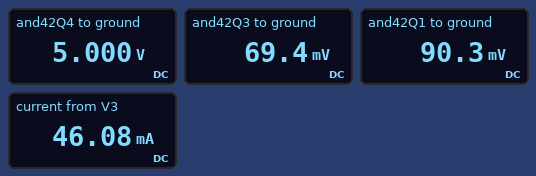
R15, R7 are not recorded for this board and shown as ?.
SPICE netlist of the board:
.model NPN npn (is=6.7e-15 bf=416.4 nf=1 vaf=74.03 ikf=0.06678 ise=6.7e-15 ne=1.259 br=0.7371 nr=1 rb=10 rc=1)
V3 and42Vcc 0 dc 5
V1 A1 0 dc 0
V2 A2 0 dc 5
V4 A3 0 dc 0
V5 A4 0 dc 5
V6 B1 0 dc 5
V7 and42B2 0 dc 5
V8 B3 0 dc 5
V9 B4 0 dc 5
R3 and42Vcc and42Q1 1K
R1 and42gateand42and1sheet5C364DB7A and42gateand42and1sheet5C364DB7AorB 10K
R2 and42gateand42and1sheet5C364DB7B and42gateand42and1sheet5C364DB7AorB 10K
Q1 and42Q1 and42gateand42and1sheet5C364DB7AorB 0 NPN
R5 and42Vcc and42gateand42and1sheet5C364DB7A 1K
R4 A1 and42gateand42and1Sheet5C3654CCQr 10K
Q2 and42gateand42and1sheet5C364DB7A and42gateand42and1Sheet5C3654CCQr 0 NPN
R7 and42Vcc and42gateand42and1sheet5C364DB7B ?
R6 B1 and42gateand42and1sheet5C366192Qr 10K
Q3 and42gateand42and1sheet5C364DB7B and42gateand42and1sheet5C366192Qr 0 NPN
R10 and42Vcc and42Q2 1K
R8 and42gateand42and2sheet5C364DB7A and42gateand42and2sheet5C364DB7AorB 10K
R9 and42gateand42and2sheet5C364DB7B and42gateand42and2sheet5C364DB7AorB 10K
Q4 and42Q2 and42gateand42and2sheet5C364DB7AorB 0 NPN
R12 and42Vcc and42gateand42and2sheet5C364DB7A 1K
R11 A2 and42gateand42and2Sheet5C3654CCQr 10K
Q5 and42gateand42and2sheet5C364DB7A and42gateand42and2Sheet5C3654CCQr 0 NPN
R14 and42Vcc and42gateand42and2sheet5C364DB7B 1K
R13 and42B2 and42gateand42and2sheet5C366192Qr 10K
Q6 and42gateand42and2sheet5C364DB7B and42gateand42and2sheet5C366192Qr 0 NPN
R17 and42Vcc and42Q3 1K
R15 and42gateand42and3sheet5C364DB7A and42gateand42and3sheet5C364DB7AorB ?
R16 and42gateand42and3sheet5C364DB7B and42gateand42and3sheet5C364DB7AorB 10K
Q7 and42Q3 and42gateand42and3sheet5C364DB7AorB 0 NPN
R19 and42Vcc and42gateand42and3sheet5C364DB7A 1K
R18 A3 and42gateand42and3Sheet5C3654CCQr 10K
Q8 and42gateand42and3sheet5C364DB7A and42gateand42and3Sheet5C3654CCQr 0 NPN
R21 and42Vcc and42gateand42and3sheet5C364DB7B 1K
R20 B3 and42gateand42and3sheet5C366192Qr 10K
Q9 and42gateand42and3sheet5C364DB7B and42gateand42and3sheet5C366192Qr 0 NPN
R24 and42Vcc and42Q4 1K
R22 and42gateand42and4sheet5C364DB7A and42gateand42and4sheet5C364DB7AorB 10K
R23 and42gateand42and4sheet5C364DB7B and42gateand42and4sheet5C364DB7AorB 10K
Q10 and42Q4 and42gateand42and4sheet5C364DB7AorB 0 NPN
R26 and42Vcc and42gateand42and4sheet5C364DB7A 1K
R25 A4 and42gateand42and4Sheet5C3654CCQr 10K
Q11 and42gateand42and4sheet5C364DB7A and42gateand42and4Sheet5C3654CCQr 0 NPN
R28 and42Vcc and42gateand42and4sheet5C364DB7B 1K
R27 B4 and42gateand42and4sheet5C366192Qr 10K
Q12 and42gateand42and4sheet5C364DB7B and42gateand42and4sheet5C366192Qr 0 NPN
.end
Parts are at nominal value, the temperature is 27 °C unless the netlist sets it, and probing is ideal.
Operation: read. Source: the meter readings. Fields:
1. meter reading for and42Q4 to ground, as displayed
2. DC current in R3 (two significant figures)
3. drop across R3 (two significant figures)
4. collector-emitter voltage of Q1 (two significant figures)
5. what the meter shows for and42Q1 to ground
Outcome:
5.000 V
4.9 mA
4.9 V
90 mV
90.3 mV
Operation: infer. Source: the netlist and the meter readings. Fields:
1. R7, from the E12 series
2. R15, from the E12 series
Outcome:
470 Ω
3.9 kΩ
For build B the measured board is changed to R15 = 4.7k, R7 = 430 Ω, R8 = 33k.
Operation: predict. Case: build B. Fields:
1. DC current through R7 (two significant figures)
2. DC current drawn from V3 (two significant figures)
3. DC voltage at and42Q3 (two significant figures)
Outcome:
11 mA
47 mA
73 mV
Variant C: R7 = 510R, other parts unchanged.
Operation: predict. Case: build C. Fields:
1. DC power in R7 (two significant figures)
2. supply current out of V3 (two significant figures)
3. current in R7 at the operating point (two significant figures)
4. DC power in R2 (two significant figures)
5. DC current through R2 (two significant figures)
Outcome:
47 mW
45 mA
9.6 mA
37 µW
61 µA
